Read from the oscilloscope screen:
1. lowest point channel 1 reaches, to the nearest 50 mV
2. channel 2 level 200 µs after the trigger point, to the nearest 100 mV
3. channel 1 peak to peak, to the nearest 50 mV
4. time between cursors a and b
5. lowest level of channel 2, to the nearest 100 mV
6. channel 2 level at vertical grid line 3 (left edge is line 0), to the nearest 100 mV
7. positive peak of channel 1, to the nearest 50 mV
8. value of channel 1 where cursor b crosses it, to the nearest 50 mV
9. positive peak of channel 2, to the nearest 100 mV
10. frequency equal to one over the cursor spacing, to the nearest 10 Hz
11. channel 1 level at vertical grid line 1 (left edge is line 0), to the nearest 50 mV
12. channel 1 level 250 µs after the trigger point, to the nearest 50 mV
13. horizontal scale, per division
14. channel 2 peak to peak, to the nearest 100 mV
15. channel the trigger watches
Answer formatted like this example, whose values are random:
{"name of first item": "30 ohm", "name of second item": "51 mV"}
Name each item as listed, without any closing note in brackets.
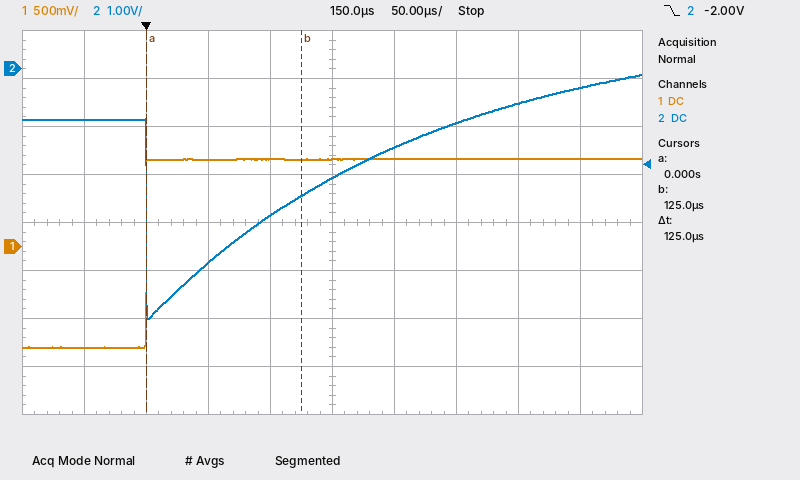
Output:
{"lowest point channel 1 reaches, to the nearest 50 mV": "-1.05 V", "channel 2 level 200 µs after the trigger point, to the nearest 100 mV": "-1.6 V", "channel 1 peak to peak, to the nearest 50 mV": "1.95 V", "time between cursors a and b": "125 µs", "lowest level of channel 2, to the nearest 100 mV": "-5.2 V", "channel 2 level at vertical grid line 3 (left edge is line 0), to the nearest 100 mV": "-4.0 V", "positive peak of channel 1, to the nearest 50 mV": "900 mV", "value of channel 1 where cursor b crosses it, to the nearest 50 mV": "900 mV", "positive peak of channel 2, to the nearest 100 mV": "-100 mV", "frequency equal to one over the cursor spacing, to the nearest 10 Hz": "8.00 kHz", "channel 1 level at vertical grid line 1 (left edge is line 0), to the nearest 50 mV": "-1.05 V", "channel 1 level 250 µs after the trigger point, to the nearest 50 mV": "900 mV", "horizontal scale, per division": "50 µs", "channel 2 peak to peak, to the nearest 100 mV": "5.1 V", "channel the trigger watches": "channel 2"}
